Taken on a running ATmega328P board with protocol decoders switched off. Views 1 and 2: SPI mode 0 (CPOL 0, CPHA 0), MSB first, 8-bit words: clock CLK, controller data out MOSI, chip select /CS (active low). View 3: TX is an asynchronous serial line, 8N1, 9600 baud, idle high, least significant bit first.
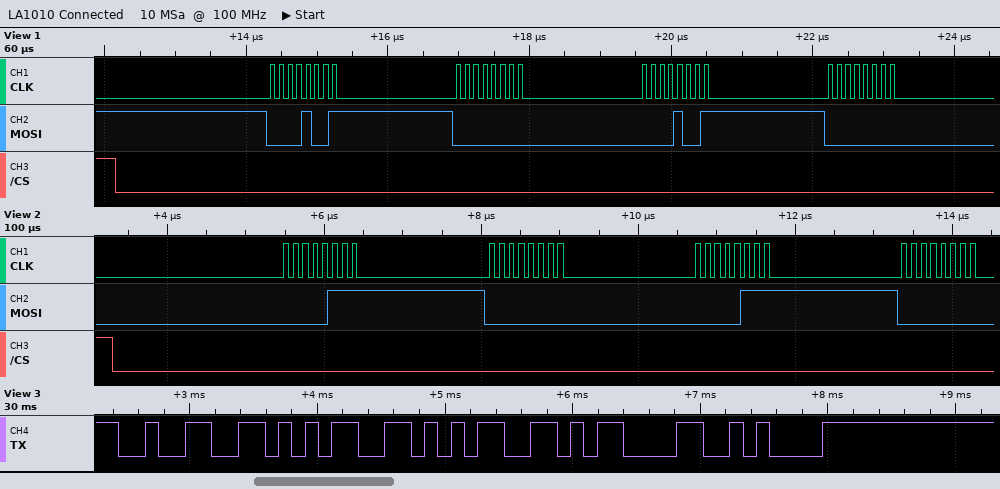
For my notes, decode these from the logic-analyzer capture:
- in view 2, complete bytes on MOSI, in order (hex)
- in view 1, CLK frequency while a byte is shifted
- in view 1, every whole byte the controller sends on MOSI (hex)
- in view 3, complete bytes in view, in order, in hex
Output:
07 00 07 00
8 MHz
09 00 09 00
32 35 35 0D 0A
